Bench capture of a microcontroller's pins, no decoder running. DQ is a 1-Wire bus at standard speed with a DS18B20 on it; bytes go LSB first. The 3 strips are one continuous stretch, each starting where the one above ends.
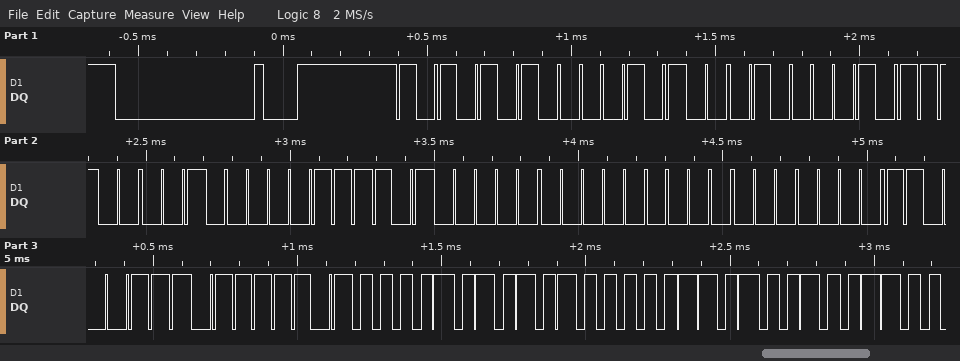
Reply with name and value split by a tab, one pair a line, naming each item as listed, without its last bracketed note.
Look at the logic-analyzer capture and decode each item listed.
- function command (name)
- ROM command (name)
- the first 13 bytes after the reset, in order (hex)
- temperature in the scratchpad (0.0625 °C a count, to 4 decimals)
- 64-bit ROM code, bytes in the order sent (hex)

function command	Read Scratchpad
ROM command	Match ROM
the first 13 bytes after the reset, in order	55 28 42 87 E0 05 00 00 E3 BE 50 05 4B
temperature in the scratchpad	85.0000 °C
64-bit ROM code, bytes in the order sent	28 42 87 E0 05 00 00 E3
